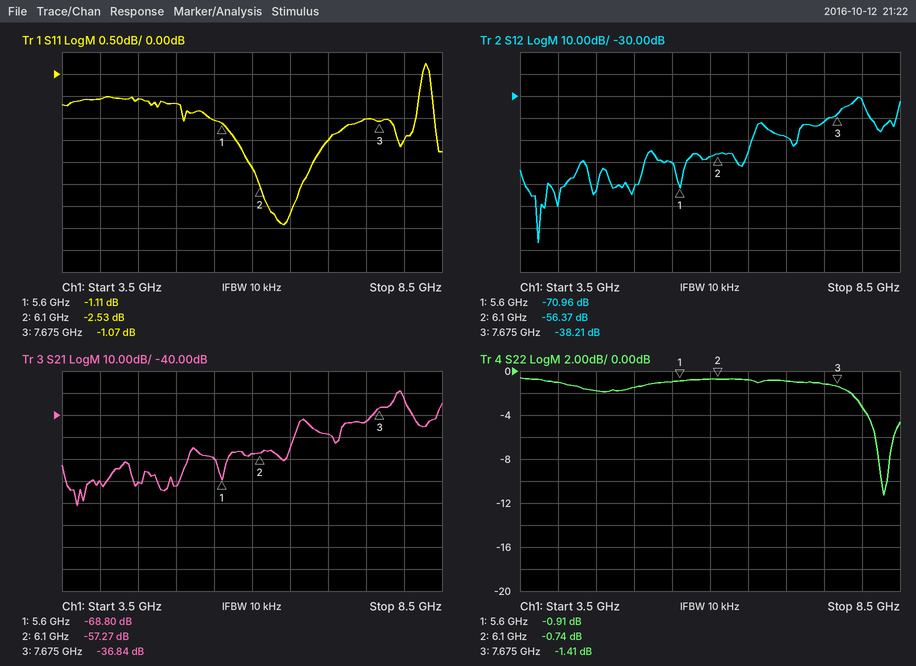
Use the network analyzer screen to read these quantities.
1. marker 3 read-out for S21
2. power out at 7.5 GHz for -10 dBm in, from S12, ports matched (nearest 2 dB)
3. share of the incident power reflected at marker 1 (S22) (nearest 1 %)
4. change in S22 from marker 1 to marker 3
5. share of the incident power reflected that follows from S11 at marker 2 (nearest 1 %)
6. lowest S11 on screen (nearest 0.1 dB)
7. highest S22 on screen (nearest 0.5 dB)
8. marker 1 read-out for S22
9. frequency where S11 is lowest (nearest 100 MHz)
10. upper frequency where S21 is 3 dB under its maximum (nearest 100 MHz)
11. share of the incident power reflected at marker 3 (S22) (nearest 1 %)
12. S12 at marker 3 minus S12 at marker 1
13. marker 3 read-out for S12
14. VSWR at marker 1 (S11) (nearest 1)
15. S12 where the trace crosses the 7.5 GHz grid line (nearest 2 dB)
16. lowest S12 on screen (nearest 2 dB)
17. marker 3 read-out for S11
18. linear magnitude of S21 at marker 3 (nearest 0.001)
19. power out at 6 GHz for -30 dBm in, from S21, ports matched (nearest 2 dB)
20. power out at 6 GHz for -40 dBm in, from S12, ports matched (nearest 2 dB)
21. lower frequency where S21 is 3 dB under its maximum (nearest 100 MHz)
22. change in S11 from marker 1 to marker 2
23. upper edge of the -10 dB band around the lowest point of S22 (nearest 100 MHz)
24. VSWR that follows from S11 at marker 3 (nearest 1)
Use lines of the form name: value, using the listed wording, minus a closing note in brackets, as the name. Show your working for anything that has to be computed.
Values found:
marker 3 read-out for S21: -36.84 dB
power out at 7.5 GHz for -10 dBm in, from S12, ports matched: -10 dBm + (-42 dB) = -52 dBm
share of the incident power reflected at marker 1 (S22): 10^(-0.91/10) ≈ 81 %
change in S22 from marker 1 to marker 3: -1.41 − (-0.91) = -0.50 dB
share of the incident power reflected that follows from S11 at marker 2: 10^(-2.53/10) ≈ 56 %
lowest S11 on screen: -3.4 dB
highest S22 on screen: -0.5 dB
marker 1 read-out for S22: -0.91 dB
frequency where S11 is lowest: 6.4 GHz
upper frequency where S21 is 3 dB under its maximum: 8.0 GHz
share of the incident power reflected at marker 3 (S22): 10^(-1.41/10) ≈ 72 %
S12 at marker 3 minus S12 at marker 1: -38.21 − (-70.96) = 32.75 dB
marker 3 read-out for S12: -38.21 dB
VSWR at marker 1 (S11): (1 + 0.8800)/(1 − 0.8800) ≈ 16
S12 where the trace crosses the 7.5 GHz grid line: -42 dB
lowest S12 on screen: -96 dB
marker 3 read-out for S11: -1.07 dB
linear magnitude of S21 at marker 3: 10^(-36.84/20) ≈ 0.014
power out at 6 GHz for -30 dBm in, from S21, ports matched: -30 dBm + (-58 dB) = -88 dBm
power out at 6 GHz for -40 dBm in, from S12, ports matched: -40 dBm + (-58 dB) = -98 dBm
lower frequency where S21 is 3 dB under its maximum: 7.9 GHz
change in S11 from marker 1 to marker 2: -2.53 − (-1.11) = -1.42 dB
upper edge of the -10 dB band around the lowest point of S22: 8.3 GHz
VSWR that follows from S11 at marker 3: (1 + 0.8841)/(1 − 0.8841) ≈ 16
